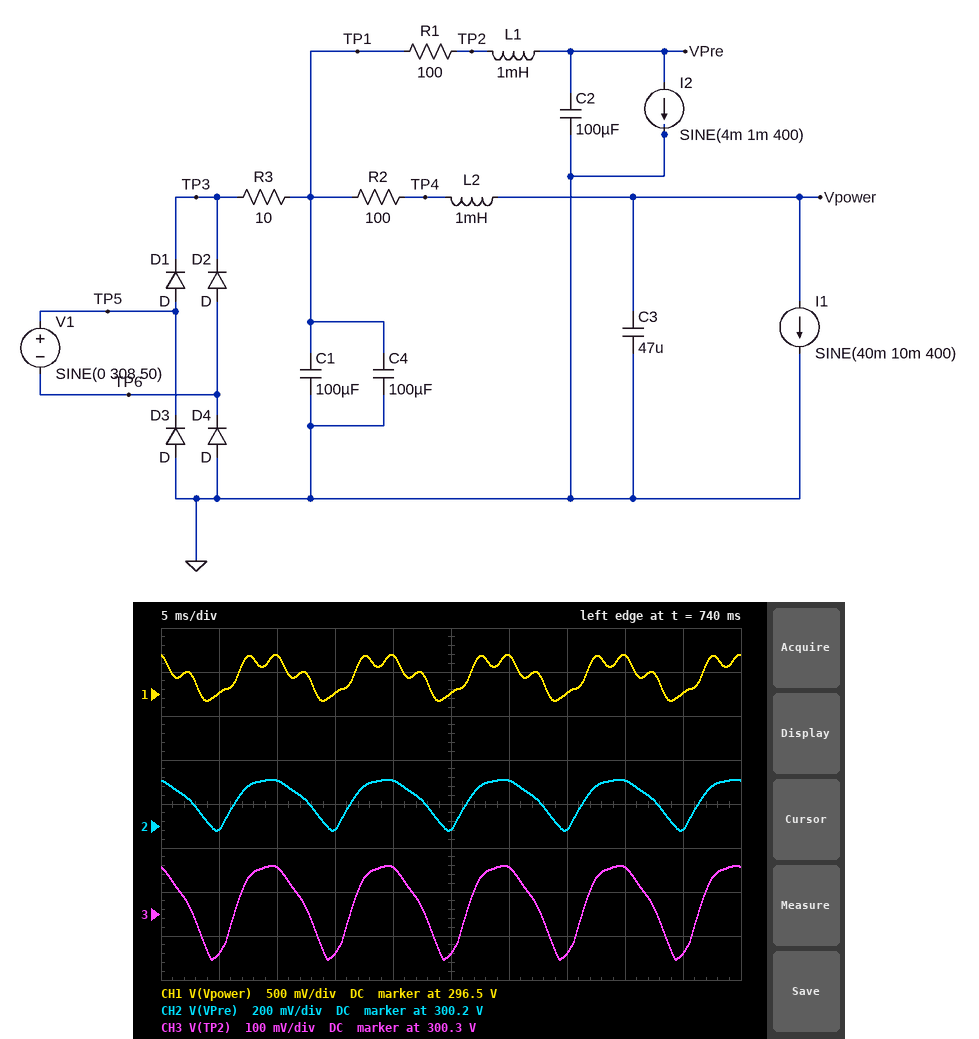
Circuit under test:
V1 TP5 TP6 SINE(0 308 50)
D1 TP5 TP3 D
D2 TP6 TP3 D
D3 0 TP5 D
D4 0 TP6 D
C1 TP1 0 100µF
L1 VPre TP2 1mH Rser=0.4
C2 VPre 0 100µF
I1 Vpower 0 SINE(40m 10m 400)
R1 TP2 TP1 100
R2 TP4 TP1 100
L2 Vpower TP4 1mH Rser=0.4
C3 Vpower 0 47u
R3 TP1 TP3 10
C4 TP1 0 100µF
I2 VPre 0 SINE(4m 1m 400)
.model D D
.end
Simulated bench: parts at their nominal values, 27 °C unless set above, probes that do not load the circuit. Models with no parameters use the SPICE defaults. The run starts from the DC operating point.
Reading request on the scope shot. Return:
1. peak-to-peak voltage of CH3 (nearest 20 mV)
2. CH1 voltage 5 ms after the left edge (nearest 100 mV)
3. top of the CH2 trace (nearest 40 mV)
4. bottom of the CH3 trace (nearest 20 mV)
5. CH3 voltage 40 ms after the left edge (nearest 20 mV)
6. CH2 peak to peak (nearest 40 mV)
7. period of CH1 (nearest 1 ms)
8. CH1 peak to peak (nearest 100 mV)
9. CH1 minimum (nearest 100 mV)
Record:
220 mV
296.5 V
300.40 V
300.20 V
300.40 V
240 mV
10 ms
500 mV
296.4 V
